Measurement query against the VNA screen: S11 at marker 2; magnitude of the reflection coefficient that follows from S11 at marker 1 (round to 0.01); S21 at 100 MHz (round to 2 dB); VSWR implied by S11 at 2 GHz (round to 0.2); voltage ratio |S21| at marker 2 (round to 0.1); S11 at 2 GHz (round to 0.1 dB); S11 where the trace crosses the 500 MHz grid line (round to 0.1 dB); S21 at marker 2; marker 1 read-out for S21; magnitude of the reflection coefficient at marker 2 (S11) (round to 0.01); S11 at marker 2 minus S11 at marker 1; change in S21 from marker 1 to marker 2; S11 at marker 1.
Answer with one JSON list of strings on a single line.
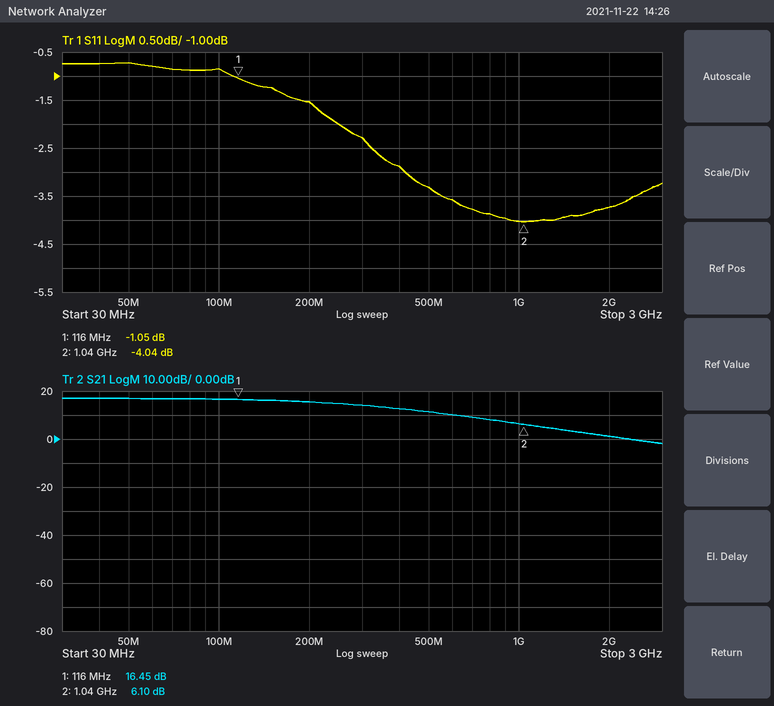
["-4.04 dB", "0.89", "16 dB", "4.8", "2.0", "-3.7 dB", "-3.3 dB", "6.10 dB", "16.45 dB", "0.63", "-2.99 dB", "-10.35 dB", "-1.05 dB"]
